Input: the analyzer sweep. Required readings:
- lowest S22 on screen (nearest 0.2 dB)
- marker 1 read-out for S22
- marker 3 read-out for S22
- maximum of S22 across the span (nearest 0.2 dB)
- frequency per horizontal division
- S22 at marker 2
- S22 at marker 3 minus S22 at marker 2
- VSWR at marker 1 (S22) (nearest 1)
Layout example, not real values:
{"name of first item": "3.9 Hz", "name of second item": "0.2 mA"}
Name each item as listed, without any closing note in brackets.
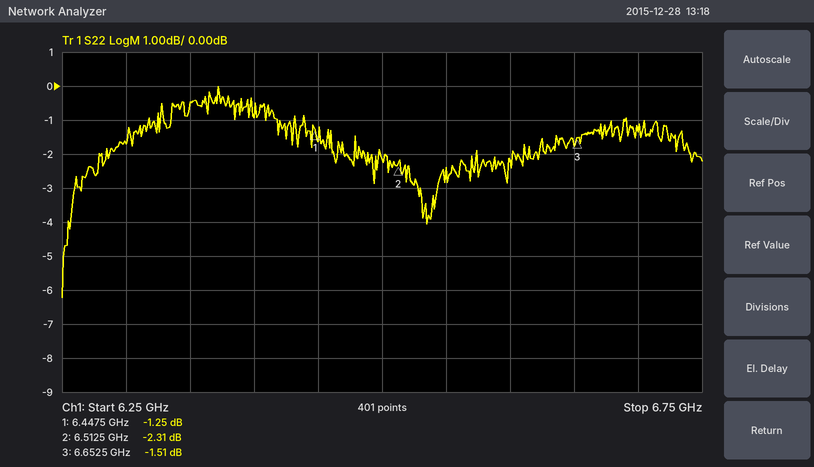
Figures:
{"lowest S22 on screen": "-6.2 dB", "marker 1 read-out for S22": "-1.25 dB", "marker 3 read-out for S22": "-1.51 dB", "maximum of S22 across the span": "0.0 dB", "frequency per horizontal division": "50 MHz", "S22 at marker 2": "-2.31 dB", "S22 at marker 3 minus S22 at marker 2": "0.80 dB", "VSWR at marker 1 (S22)": "14"}
